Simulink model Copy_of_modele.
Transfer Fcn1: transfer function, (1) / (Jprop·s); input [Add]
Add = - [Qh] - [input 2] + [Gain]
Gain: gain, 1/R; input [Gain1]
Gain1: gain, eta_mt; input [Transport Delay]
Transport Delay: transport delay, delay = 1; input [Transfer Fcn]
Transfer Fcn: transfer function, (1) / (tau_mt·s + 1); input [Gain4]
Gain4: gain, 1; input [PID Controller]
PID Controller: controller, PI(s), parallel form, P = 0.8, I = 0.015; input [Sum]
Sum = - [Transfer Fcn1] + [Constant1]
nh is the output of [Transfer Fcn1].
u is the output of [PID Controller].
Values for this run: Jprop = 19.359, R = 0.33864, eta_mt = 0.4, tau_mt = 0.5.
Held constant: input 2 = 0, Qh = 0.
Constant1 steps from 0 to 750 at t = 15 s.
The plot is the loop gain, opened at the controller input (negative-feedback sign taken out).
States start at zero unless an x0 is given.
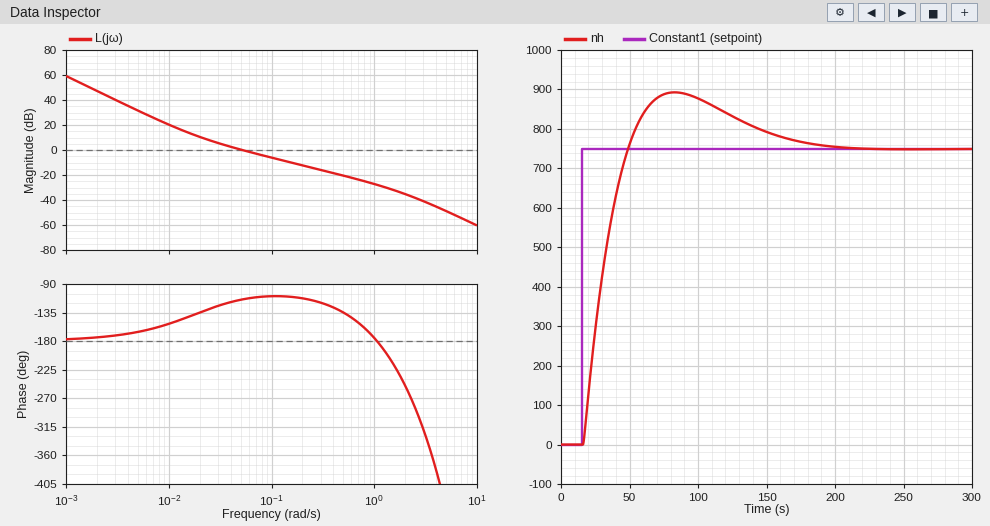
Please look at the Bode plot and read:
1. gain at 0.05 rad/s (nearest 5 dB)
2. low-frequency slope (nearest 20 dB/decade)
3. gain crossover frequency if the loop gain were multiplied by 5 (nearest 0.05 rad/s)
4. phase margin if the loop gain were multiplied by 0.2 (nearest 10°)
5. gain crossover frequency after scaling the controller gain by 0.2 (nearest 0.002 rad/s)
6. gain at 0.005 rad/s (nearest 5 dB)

0 dB
-40 dB/decade
0.25 rad/s
40°
0.016 rad/s
30 dB
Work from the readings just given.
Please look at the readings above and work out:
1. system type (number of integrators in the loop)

2
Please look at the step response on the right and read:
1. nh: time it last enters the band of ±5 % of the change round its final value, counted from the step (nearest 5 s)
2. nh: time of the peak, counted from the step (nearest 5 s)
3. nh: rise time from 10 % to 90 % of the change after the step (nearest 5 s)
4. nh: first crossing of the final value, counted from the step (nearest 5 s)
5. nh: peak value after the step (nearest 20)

140 s
70 s
25 s
35 s
900
